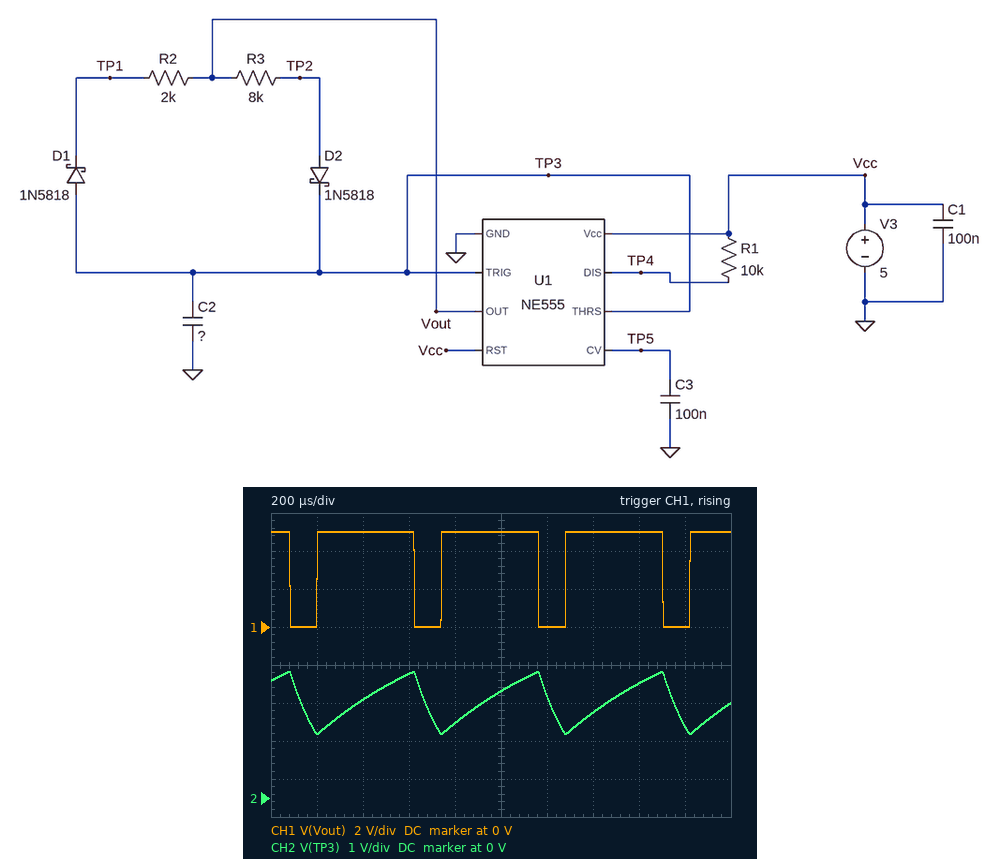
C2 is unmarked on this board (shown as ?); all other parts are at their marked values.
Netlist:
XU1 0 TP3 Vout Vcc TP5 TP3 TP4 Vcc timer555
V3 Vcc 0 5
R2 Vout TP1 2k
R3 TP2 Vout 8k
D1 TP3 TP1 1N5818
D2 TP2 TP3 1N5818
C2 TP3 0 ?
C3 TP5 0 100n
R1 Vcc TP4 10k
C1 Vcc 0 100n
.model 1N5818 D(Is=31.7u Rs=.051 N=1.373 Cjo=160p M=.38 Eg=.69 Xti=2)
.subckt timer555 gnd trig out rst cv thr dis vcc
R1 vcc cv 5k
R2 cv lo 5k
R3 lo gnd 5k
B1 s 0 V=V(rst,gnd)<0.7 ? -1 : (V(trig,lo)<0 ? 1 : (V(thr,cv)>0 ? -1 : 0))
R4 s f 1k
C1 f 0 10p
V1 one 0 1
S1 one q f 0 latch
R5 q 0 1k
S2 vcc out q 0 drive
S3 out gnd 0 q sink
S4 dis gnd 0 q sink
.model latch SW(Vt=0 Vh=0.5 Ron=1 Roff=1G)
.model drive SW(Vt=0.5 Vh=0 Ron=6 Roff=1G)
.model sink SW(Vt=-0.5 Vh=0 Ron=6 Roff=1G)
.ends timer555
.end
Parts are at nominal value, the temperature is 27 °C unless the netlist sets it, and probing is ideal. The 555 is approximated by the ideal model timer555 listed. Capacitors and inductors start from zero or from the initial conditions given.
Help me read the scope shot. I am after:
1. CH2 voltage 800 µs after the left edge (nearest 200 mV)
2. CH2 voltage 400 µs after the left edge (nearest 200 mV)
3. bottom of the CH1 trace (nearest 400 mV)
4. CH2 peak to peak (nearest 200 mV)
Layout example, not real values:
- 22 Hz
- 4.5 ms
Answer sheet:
- 2.0 V
- 2.6 V
- 0 V
- 1.6 V
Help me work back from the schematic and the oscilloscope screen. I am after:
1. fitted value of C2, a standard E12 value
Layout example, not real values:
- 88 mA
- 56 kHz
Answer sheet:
- 82 nF
